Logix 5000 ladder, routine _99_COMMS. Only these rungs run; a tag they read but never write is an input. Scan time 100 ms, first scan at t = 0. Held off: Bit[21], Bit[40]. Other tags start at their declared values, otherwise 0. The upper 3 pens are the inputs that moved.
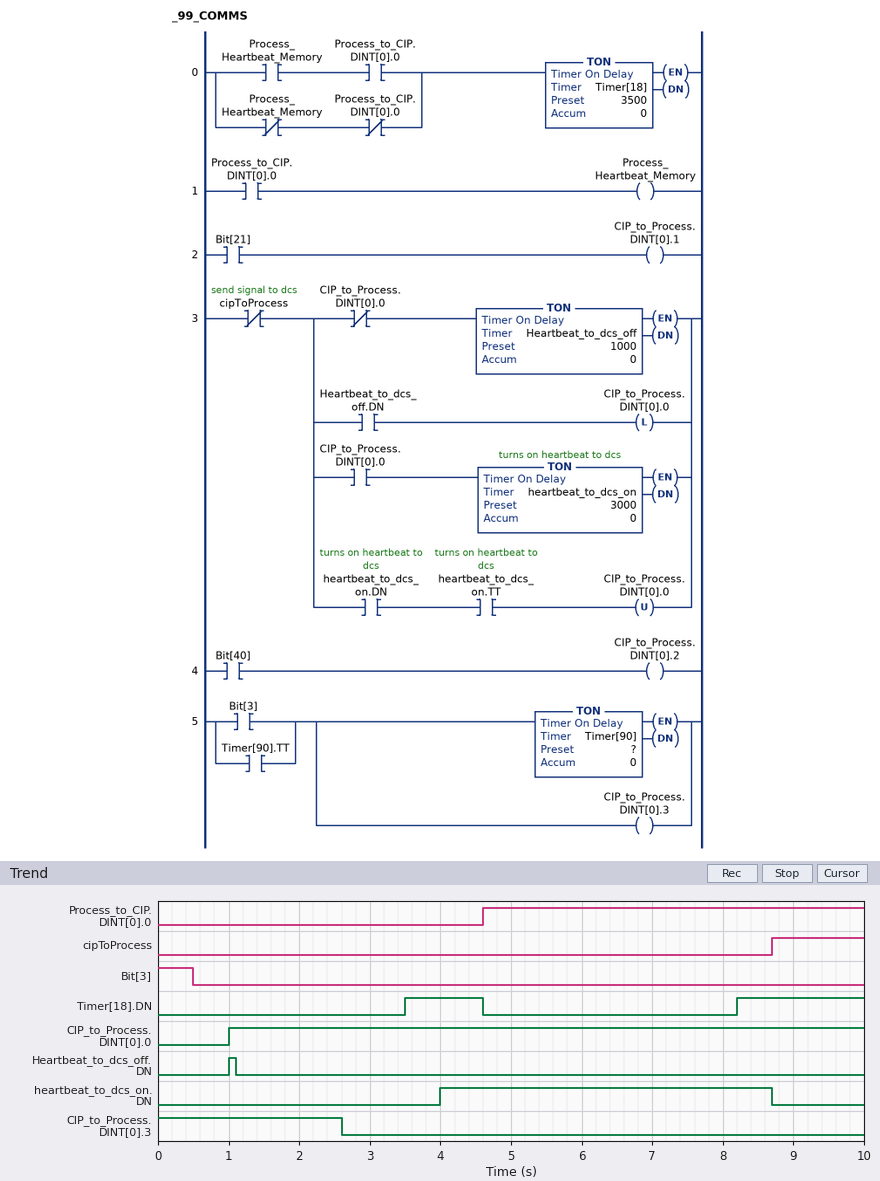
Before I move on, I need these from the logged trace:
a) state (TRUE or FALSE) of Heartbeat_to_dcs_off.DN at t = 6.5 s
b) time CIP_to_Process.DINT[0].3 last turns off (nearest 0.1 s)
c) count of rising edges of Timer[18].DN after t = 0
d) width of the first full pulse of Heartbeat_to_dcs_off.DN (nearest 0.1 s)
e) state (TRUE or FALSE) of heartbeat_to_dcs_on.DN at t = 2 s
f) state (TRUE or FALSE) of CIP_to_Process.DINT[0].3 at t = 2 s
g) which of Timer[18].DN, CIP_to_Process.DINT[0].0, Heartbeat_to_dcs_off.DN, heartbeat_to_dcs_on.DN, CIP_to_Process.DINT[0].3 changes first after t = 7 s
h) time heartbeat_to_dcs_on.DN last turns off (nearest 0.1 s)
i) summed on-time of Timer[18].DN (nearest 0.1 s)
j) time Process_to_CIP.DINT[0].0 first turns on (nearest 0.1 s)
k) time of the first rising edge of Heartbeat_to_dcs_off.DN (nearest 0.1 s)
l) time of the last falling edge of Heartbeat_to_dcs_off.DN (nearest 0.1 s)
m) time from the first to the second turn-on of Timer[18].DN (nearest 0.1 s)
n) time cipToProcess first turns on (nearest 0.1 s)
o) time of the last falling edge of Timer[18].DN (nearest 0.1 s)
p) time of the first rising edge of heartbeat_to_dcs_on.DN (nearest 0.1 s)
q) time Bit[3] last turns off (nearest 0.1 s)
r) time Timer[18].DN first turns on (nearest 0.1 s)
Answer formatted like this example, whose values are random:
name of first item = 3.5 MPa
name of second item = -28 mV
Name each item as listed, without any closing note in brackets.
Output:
state (TRUE or FALSE) of Heartbeat_to_dcs_off.DN at t = 6.5 s = FALSE
time CIP_to_Process.DINT[0].3 last turns off = 2.6 s
count of rising edges of Timer[18].DN after t = 0 = 2
width of the first full pulse of Heartbeat_to_dcs_off.DN = 0.1 s
state (TRUE or FALSE) of heartbeat_to_dcs_on.DN at t = 2 s = FALSE
state (TRUE or FALSE) of CIP_to_Process.DINT[0].3 at t = 2 s = TRUE
which of Timer[18].DN, CIP_to_Process.DINT[0].0, Heartbeat_to_dcs_off.DN, heartbeat_to_dcs_on.DN, CIP_to_Process.DINT[0].3 changes first after t = 7 s = Timer[18].DN
time heartbeat_to_dcs_on.DN last turns off = 8.7 s
summed on-time of Timer[18].DN = 2.9 s
time Process_to_CIP.DINT[0].0 first turns on = 4.6 s
time of the first rising edge of Heartbeat_to_dcs_off.DN = 1.0 s
time of the last falling edge of Heartbeat_to_dcs_off.DN = 1.1 s
time from the first to the second turn-on of Timer[18].DN = 4.7 s
time cipToProcess first turns on = 8.7 s
time of the last falling edge of Timer[18].DN = 4.6 s
time of the first rising edge of heartbeat_to_dcs_on.DN = 4.0 s
time Bit[3] last turns off = 0.5 s
time Timer[18].DN first turns on = 3.5 s
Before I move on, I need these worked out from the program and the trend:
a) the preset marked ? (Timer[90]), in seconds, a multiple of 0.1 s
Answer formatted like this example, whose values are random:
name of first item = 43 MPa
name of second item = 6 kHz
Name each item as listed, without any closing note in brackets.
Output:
the preset marked ? (Timer[90]), in seconds, a multiple of 0.1 s = 2.5 s
